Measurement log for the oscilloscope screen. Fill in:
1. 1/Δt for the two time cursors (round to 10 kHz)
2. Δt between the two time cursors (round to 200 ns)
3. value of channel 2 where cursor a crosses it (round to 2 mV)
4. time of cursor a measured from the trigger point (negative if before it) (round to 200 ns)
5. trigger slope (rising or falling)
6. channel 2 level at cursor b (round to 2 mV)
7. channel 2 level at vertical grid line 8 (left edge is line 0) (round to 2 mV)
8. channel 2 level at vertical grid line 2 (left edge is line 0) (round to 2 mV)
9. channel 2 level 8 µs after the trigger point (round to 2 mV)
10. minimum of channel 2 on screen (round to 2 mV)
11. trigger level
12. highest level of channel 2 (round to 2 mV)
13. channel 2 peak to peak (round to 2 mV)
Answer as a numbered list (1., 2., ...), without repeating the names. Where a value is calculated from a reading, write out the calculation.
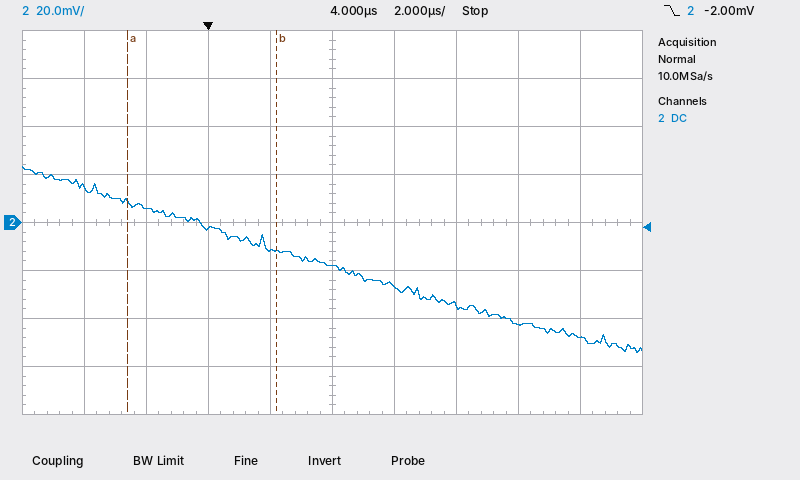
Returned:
1. 1 / 4.8 µs ≈ 210 kHz
2. 4.8 µs
3. 8 mV
4. -2.6 µs
5. falling
6. -12 mV
7. -42 mV
8. 6 mV
9. -34 mV
10. -54 mV
11. -2.00 mV
12. 24 mV
13. 24 mV − (-54 mV) = 78 mV
